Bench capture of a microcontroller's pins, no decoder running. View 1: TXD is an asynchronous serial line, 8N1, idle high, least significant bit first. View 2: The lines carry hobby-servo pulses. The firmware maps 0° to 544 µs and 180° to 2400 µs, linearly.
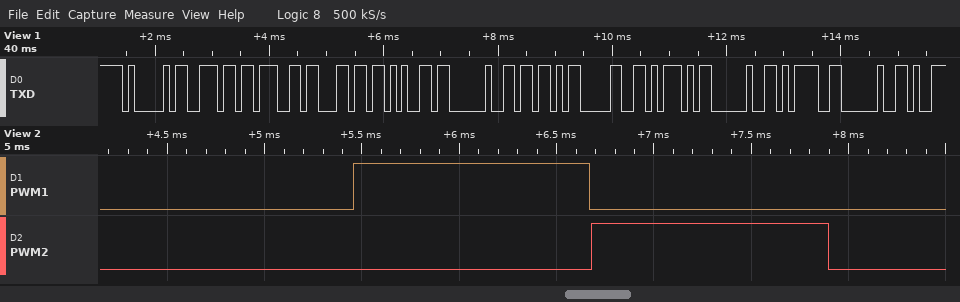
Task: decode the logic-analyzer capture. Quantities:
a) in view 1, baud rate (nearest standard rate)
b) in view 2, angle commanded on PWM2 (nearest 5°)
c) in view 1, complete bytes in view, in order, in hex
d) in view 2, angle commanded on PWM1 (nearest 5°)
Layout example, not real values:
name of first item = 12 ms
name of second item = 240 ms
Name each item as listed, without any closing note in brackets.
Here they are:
in view 1, baud rate = 9600 baud
in view 2, angle commanded on PWM2 = 65°
in view 1, complete bytes in view, in order, in hex = 41 6E 67 6C 65 20 5B 30 5D 20 3D 20
in view 2, angle commanded on PWM1 = 65°
